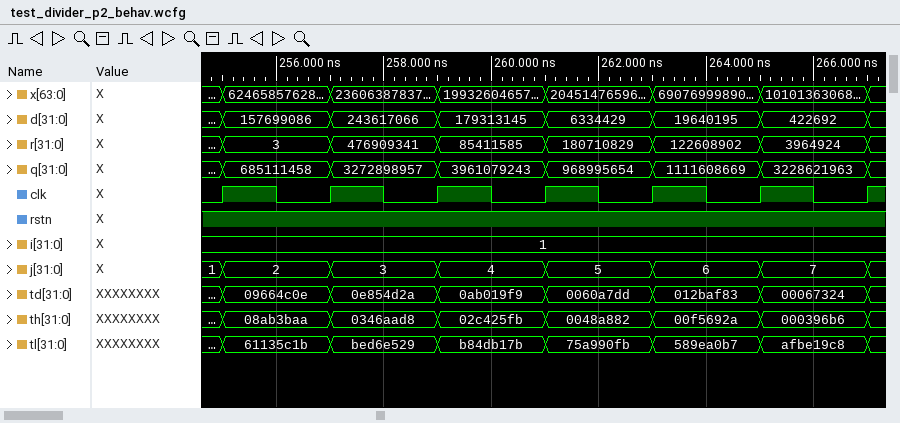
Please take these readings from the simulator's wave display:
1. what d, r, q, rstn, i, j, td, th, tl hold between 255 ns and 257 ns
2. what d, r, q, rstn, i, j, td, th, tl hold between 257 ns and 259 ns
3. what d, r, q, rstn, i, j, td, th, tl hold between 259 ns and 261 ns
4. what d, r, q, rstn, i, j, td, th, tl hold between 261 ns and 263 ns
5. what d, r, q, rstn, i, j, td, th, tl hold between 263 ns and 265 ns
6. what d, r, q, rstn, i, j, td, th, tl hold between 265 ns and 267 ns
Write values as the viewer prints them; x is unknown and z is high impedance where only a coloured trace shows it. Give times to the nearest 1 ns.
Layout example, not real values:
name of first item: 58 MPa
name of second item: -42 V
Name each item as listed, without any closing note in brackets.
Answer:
what d, r, q, rstn, i, j, td, th, tl hold between 255 ns and 257 ns: d=157699086, r=3, q=685111458, rstn=1, i=1, j=2, td=09664c0e, th=08ab3baa, tl=61135c1b
what d, r, q, rstn, i, j, td, th, tl hold between 257 ns and 259 ns: d=243617066, r=476909341, q=3272898957, rstn=1, i=1, j=3, td=0e854d2a, th=0346aad8, tl=bed6e529
what d, r, q, rstn, i, j, td, th, tl hold between 259 ns and 261 ns: d=179313145, r=85411585, q=3961079243, rstn=1, i=1, j=4, td=0ab019f9, th=02c425fb, tl=b84db17b
what d, r, q, rstn, i, j, td, th, tl hold between 261 ns and 263 ns: d=6334429, r=180710829, q=968995654, rstn=1, i=1, j=5, td=0060a7dd, th=0048a882, tl=75a990fb
what d, r, q, rstn, i, j, td, th, tl hold between 263 ns and 265 ns: d=19640195, r=122608902, q=1111608669, rstn=1, i=1, j=6, td=012baf83, th=00f5692a, tl=589ea0b7
what d, r, q, rstn, i, j, td, th, tl hold between 265 ns and 267 ns: d=422692, r=3964924, q=3228621963, rstn=1, i=1, j=7, td=00067324, th=000396b6, tl=afbe19c8
